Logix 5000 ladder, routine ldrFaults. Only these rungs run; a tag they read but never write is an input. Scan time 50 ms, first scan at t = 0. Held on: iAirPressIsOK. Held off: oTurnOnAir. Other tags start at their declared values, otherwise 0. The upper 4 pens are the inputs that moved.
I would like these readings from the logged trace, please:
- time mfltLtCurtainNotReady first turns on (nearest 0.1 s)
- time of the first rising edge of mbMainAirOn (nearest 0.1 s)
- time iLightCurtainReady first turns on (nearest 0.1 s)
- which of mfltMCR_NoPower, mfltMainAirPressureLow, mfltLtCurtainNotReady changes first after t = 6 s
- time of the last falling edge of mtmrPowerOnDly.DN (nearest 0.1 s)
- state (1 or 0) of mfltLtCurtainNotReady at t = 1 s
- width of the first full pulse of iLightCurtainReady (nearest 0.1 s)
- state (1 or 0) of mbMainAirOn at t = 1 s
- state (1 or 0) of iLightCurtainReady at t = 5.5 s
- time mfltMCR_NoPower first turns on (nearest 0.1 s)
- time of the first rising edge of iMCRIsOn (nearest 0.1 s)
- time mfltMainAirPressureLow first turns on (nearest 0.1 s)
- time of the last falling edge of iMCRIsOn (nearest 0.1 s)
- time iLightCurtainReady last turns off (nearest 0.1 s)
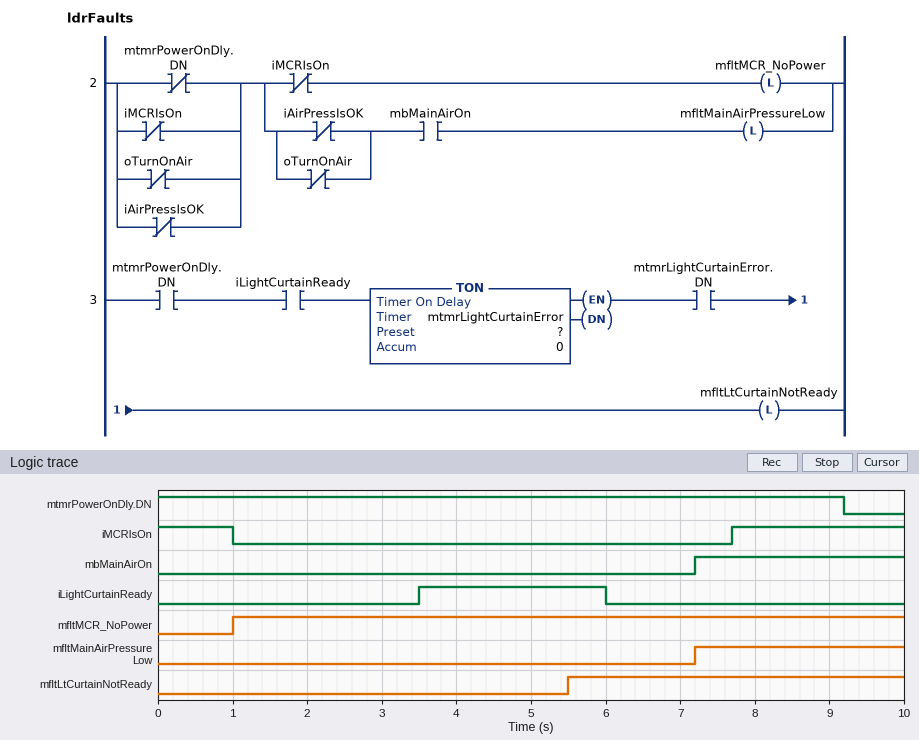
5.5 s
7.2 s
3.5 s
mfltMainAirPressureLow
9.2 s
0
2.5 s
0
1
1.0 s
7.7 s
7.2 s
1.0 s
6.0 s
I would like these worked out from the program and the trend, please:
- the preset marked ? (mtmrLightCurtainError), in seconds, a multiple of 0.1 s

2.0 s
